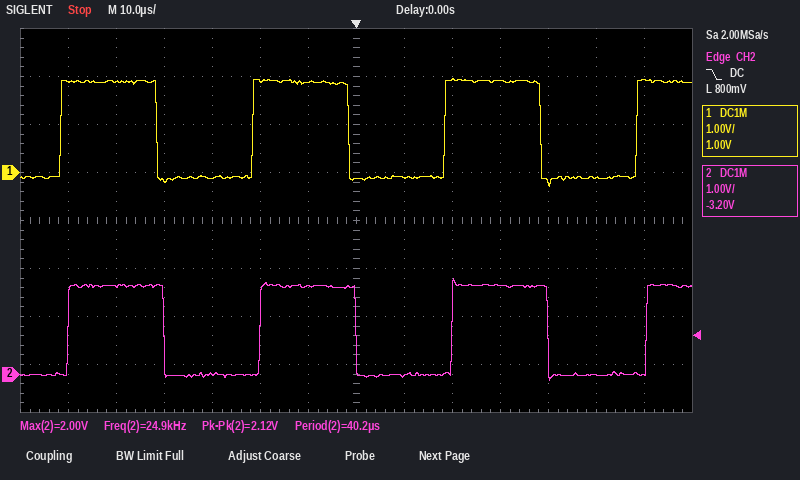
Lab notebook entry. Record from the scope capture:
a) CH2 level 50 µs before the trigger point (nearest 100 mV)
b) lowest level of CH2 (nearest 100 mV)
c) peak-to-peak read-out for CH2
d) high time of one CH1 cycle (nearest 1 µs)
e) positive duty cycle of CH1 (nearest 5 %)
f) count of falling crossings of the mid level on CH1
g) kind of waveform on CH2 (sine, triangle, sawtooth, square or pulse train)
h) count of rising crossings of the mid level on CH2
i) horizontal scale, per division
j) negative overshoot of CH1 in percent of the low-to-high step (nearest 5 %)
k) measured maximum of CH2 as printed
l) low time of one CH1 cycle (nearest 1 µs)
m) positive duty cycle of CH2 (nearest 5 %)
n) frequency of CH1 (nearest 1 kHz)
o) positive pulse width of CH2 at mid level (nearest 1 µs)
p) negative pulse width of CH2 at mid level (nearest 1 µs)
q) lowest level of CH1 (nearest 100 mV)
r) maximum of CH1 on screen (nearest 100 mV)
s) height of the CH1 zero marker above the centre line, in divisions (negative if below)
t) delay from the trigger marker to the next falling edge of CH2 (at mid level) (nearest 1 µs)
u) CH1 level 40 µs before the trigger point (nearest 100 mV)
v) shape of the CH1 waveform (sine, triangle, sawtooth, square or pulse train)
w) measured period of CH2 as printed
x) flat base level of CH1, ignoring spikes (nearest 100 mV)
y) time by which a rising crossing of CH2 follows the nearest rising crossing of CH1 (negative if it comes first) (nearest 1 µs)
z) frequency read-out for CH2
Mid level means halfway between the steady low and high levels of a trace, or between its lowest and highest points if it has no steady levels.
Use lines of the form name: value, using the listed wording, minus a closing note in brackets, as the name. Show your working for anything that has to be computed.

CH2 level 50 µs before the trigger point: 1.8 V
lowest level of CH2: -100 mV
peak-to-peak read-out for CH2: 2.12 V
high time of one CH1 cycle: 20 µs
positive duty cycle of CH1: 20 µs / 40 µs ≈ 50 %
count of falling crossings of the mid level on CH1: 3
kind of waveform on CH2: square
count of rising crossings of the mid level on CH2: 4
horizontal scale, per division: 10 µs
negative overshoot of CH1 in percent of the low-to-high step: 10 %
measured maximum of CH2 as printed: 2.00 V
low time of one CH1 cycle: 20 µs
positive duty cycle of CH2: 50 %
frequency of CH1: 1 / 40 µs ≈ 25 kHz
positive pulse width of CH2 at mid level: 20 µs
negative pulse width of CH2 at mid level: 20 µs
lowest level of CH1: -300 mV
maximum of CH1 on screen: 2.0 V
height of the CH1 zero marker above the centre line, in divisions: +1.0 div
delay from the trigger marker to the next falling edge of CH2 (at mid level): 40 µs
CH1 level 40 µs before the trigger point: -200 mV
shape of the CH1 waveform: square
measured period of CH2 as printed: 40.2 µs
flat base level of CH1, ignoring spikes: -100 mV
time by which a rising crossing of CH2 follows the nearest rising crossing of CH1 (negative if it comes first): +2 µs
frequency read-out for CH2: 24.9 kHz
